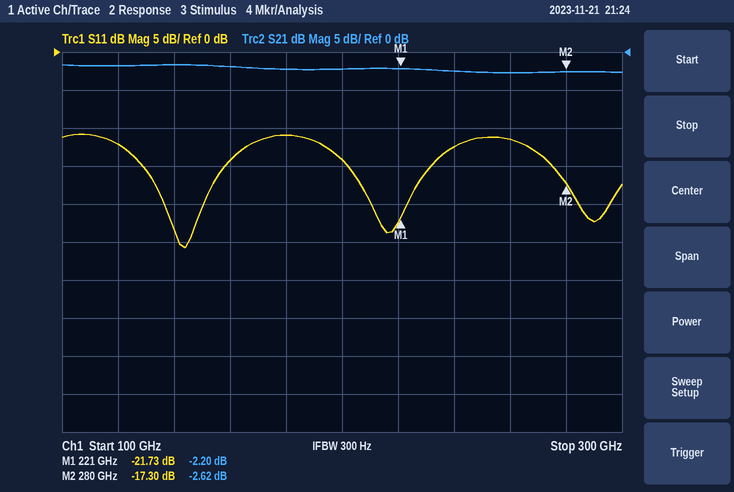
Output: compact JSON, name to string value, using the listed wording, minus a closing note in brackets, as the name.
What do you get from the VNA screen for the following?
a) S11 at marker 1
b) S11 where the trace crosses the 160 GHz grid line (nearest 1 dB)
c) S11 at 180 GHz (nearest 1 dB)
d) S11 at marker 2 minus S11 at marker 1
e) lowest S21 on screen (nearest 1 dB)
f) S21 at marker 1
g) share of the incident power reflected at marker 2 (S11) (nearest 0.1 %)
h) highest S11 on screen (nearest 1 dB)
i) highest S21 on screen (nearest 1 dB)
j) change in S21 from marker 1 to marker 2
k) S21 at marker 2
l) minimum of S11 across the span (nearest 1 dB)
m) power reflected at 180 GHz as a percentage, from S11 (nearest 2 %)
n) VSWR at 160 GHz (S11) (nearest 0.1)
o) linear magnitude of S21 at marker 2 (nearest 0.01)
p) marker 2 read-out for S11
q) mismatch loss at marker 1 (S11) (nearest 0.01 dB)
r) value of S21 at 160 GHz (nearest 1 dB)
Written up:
{"S11 at marker 1": "-21.73 dB", "S11 where the trace crosses the 160 GHz grid line": "-14 dB", "S11 at 180 GHz": "-11 dB", "S11 at marker 2 minus S11 at marker 1": "4.43 dB", "lowest S21 on screen": "-3 dB", "S21 at marker 1": "-2.20 dB", "share of the incident power reflected at marker 2 (S11)": "1.9 %", "highest S11 on screen": "-11 dB", "highest S21 on screen": "-2 dB", "change in S21 from marker 1 to marker 2": "-0.42 dB", "S21 at marker 2": "-2.62 dB", "minimum of S11 across the span": "-26 dB", "power reflected at 180 GHz as a percentage, from S11": "8 %", "VSWR at 160 GHz (S11)": "1.5", "linear magnitude of S21 at marker 2": "0.74", "marker 2 read-out for S11": "-17.30 dB", "mismatch loss at marker 1 (S11)": "0.03 dB", "value of S21 at 160 GHz": "-2 dB"}
